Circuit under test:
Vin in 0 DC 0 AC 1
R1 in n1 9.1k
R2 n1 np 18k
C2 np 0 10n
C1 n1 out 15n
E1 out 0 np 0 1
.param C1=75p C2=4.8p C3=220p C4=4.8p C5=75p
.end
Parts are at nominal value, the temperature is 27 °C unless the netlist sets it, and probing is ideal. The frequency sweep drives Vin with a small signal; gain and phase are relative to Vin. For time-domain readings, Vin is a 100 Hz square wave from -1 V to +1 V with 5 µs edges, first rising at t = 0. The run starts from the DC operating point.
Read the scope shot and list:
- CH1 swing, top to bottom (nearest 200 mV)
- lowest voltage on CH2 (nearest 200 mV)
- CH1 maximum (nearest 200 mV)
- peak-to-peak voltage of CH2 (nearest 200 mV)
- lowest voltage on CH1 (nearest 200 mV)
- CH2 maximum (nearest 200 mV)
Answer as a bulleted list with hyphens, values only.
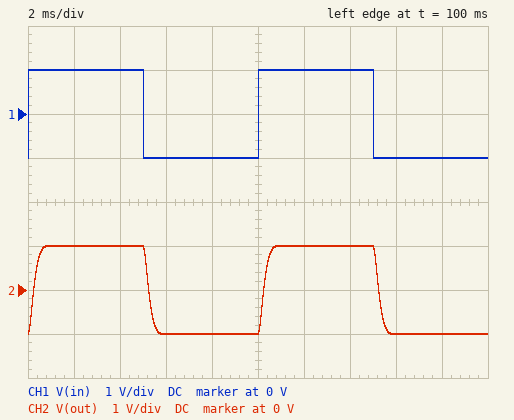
- 2.0 V
- -1.0 V
- 1.0 V
- 2.0 V
- -1.0 V
- 1.0 V
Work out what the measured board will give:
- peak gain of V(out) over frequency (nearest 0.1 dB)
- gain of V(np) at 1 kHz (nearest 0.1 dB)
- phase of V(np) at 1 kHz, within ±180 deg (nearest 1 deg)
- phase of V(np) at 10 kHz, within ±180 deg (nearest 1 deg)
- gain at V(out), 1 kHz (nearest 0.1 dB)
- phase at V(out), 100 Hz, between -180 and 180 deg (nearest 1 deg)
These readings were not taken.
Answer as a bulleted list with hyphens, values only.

- 0 dB
- -4.6 dB
- -89 deg
- -170 deg
- -4.6 dB
- -10 deg
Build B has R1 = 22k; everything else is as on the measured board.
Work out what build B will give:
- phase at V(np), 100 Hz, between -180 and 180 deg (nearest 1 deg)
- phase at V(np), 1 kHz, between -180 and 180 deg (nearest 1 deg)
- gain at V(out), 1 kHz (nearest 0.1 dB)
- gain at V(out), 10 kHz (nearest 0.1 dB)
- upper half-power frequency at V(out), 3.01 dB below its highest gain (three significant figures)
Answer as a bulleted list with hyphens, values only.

- -14 deg
- -118 deg
- -9.1 dB
- -47.4 dB
- 551 Hz
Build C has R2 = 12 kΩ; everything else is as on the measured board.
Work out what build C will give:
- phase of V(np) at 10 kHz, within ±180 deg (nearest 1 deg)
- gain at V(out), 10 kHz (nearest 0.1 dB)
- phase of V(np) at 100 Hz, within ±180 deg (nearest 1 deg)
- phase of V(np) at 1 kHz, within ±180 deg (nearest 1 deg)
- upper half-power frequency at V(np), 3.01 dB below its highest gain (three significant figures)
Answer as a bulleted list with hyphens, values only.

- -168 deg
- -36.3 dB
- -8 deg
- -75 deg
- 1.04 kHz
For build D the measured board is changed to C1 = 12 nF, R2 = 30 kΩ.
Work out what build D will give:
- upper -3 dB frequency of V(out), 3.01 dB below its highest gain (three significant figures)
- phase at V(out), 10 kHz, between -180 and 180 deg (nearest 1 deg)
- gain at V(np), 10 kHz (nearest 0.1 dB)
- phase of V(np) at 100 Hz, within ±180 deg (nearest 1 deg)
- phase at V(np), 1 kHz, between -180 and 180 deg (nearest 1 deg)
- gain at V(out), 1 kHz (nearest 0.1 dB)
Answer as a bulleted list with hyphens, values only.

- 508 Hz
- -169 deg
- -42.3 dB
- -14 deg
- -97 deg
- -7.9 dB
